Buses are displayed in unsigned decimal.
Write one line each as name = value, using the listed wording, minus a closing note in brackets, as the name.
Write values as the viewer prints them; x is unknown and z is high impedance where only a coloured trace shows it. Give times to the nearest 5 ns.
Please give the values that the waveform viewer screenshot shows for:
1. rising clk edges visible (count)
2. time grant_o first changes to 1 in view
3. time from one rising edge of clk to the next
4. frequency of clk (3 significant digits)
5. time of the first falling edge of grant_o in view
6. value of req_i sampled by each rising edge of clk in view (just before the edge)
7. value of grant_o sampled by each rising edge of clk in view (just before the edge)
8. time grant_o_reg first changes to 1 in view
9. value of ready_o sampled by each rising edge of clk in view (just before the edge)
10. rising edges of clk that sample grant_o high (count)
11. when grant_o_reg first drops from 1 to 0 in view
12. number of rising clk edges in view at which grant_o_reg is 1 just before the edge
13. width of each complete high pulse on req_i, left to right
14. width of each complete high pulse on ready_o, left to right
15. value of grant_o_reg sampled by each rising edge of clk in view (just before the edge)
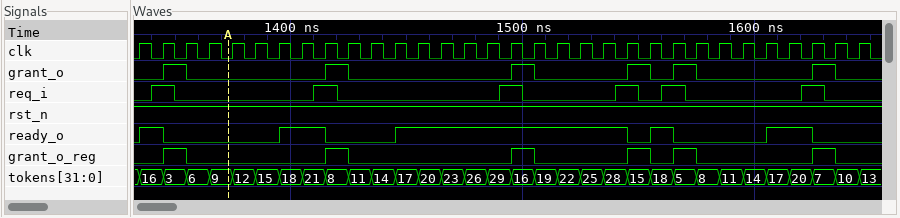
rising clk edges visible = 32
time grant_o first changes to 1 in view = 1345 ns
time from one rising edge of clk to the next = 10 ns
frequency of clk = 100 MHz
time of the first falling edge of grant_o in view = 1355 ns
value of req_i sampled by each rising edge of clk in view = 0 1 0 0 0 0 0 0 1 0 0 0 0 0 0 0 1 0 0 0 0 1 0 1 0 0 0 0 0 1 0 0
value of grant_o sampled by each rising edge of clk in view = 0 0 1 0 0 0 0 0 0 1 0 0 0 0 0 0 0 1 0 0 0 0 1 0 1 0 0 0 0 0 1 0
time grant_o_reg first changes to 1 in view = 1345 ns
value of ready_o sampled by each rising edge of clk in view = 0 1 0 0 0 0 0 1 1 0 0 0 1 1 1 1 1 1 1 1 1 1 0 1 0 0 0 0 1 1 0 0
rising edges of clk that sample grant_o high = 6
when grant_o_reg first drops from 1 to 0 in view = 1355 ns
number of rising clk edges in view at which grant_o_reg is 1 just before the edge = 6
width of each complete high pulse on req_i, left to right = 10 ns, 10 ns, 10 ns, 10 ns, 10 ns, 10 ns
width of each complete high pulse on ready_o, left to right = 10 ns, 20 ns, 100 ns, 10 ns, 20 ns
value of grant_o_reg sampled by each rising edge of clk in view = 0 0 1 0 0 0 0 0 0 1 0 0 0 0 0 0 0 1 0 0 0 0 1 0 1 0 0 0 0 0 1 0
